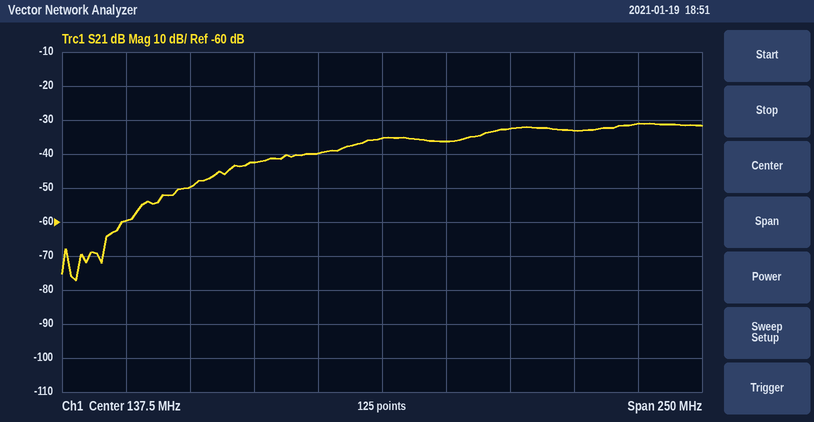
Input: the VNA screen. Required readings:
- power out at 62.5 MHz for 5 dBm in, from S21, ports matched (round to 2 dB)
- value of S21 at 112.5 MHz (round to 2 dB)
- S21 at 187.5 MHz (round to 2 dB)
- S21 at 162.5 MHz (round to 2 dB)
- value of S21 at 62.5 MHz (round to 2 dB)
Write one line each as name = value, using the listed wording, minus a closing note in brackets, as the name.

power out at 62.5 MHz for 5 dBm in, from S21, ports matched = -44 dBm
value of S21 at 112.5 MHz = -40 dB
S21 at 187.5 MHz = -32 dB
S21 at 162.5 MHz = -36 dB
value of S21 at 62.5 MHz = -50 dB
